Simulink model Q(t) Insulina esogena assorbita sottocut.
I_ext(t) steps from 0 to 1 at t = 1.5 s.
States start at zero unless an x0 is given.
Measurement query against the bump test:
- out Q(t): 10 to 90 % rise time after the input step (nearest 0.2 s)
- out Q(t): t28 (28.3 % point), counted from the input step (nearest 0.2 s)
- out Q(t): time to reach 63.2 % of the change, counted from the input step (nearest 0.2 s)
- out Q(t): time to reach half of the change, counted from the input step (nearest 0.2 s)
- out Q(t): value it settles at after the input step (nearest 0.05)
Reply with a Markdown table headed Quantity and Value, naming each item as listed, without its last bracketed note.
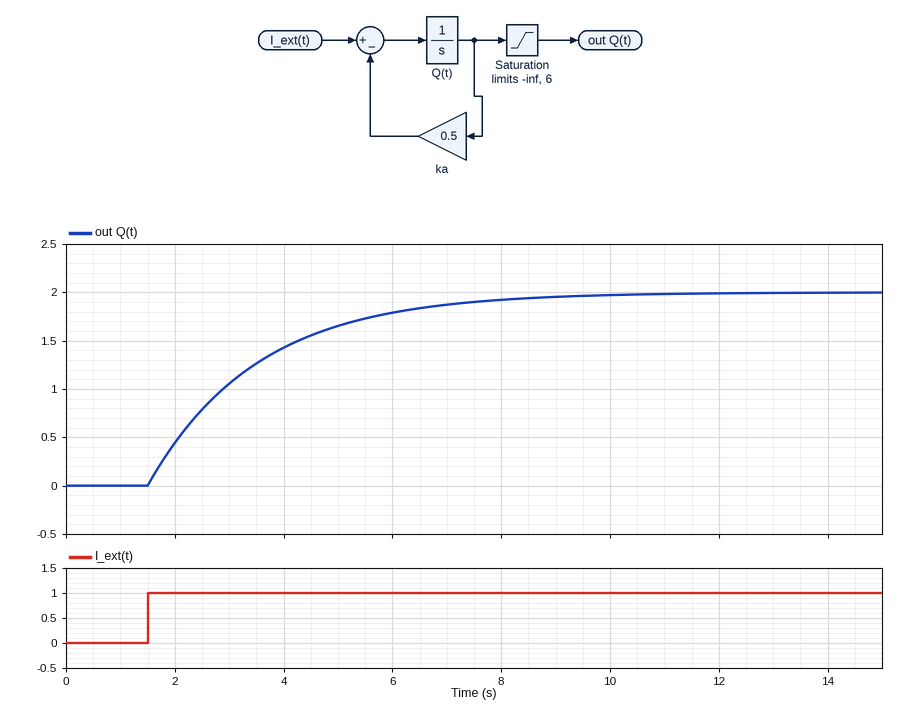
| Quantity | Value |
|---|---|
| out Q(t): 10 to 90 % rise time after the input step | 4.4 s |
| out Q(t): t28 (28.3 % point), counted from the input step | 0.6 s |
| out Q(t): time to reach 63.2 % of the change, counted from the input step | 2.0 s |
| out Q(t): time to reach half of the change, counted from the input step | 1.4 s |
| out Q(t): value it settles at after the input step | 2.00 |
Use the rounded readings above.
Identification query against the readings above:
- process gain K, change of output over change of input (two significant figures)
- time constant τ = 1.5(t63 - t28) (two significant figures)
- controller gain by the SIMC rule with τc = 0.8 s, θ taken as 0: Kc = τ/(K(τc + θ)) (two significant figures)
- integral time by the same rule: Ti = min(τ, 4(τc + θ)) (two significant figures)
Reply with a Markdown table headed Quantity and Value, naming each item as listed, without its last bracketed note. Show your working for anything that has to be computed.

| Quantity | Value |
|---|---|
| process gain K, change of output over change of input | (2 - 0) / 1 = 2.0 |
| time constant τ = 1.5(t63 - t28) | 1.5 × (2 - 0.6) = 2.1 s |
| controller gain by the SIMC rule with τc = 0.8 s, θ taken as 0: Kc = τ/(K(τc + θ)) | 2.1 / (2 × (0.8 + 0)) = 1.3 |
| integral time by the same rule: Ti = min(τ, 4(τc + θ)) | min(2.1, 4 × (0.8 + 0)) = 2.1 s |
